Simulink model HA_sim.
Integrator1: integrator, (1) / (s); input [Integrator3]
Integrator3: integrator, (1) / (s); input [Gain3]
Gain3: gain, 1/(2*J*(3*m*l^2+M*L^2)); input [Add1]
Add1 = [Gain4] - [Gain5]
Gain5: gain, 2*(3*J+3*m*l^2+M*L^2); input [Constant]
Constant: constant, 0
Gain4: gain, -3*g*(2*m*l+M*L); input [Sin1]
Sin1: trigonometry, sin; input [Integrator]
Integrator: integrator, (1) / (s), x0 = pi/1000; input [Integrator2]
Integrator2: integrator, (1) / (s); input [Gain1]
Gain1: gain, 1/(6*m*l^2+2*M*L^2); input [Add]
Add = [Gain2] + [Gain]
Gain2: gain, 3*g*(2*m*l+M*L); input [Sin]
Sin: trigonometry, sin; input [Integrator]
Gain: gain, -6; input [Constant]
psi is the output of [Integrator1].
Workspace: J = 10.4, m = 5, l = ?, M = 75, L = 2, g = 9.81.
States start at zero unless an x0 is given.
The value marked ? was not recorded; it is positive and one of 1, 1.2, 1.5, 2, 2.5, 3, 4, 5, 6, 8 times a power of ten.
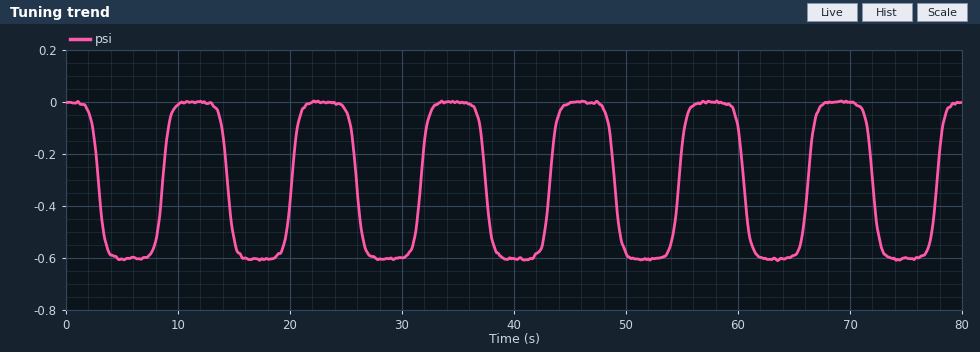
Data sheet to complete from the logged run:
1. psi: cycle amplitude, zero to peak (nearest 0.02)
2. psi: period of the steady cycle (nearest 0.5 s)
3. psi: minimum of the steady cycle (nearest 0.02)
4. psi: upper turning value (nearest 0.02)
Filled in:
0.30
11.5 s
-0.60
0.00
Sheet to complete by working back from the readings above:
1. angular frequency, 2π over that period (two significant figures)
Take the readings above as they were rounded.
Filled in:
0.55 rad/s
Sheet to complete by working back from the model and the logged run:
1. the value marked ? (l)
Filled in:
1.2
